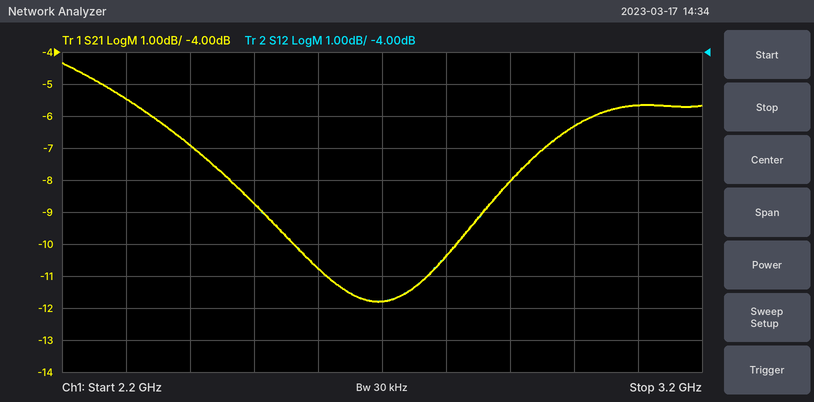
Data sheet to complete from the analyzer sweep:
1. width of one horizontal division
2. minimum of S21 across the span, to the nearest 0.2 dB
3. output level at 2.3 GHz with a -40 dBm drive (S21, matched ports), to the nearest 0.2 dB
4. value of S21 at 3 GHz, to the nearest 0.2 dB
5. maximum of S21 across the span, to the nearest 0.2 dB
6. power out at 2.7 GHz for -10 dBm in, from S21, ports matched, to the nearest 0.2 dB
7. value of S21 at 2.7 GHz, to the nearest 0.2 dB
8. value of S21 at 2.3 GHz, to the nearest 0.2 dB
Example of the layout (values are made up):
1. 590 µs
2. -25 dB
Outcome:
1. 100 MHz
2. -11.8 dB
3. -45.4 dBm
4. -6.4 dB
5. -4.4 dB
6. -21.8 dBm
7. -11.8 dB
8. -5.4 dB
